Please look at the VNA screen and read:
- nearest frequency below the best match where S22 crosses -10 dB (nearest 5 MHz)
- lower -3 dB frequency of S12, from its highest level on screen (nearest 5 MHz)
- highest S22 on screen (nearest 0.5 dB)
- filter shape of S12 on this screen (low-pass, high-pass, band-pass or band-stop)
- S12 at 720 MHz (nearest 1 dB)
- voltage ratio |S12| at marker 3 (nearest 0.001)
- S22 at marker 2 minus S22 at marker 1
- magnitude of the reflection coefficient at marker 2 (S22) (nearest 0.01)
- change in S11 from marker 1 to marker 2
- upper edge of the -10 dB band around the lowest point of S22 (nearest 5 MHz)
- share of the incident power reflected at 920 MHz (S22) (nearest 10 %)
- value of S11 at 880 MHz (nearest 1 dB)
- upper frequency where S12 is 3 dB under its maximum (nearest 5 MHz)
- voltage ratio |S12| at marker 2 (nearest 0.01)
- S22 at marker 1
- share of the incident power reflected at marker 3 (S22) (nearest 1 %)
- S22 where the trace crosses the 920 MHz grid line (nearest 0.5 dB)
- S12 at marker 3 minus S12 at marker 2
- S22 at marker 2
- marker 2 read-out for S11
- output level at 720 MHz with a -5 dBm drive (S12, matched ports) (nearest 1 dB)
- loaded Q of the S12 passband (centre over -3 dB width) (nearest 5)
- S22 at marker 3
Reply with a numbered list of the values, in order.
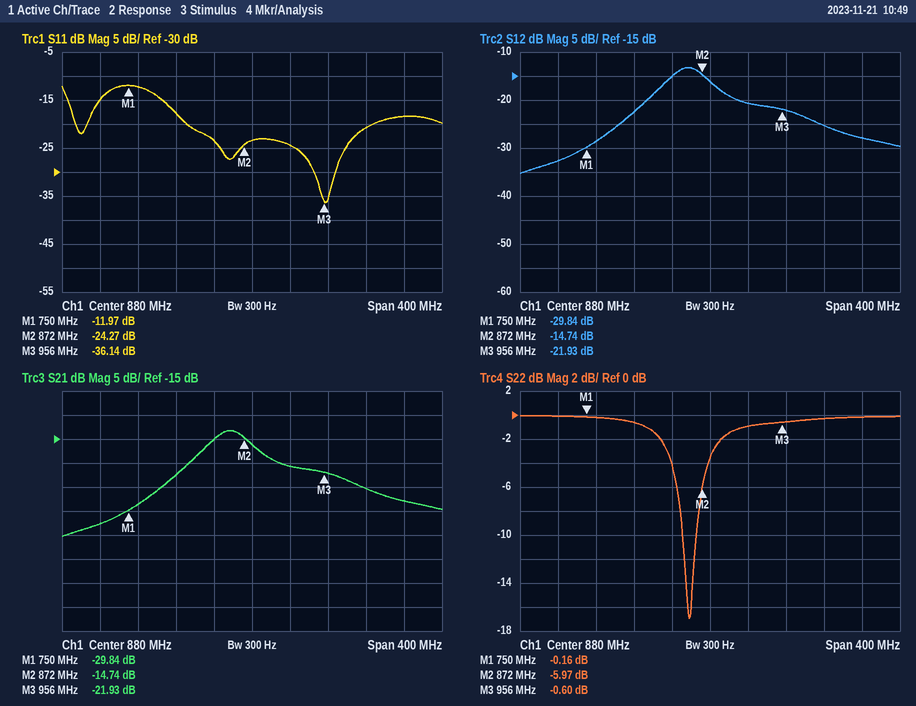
1. 850 MHz
2. 835 MHz
3. 0.0 dB
4. band-pass
5. -33 dB
6. 0.080
7. -5.81 dB
8. 0.50
9. -12.30 dB
10. 865 MHz
11. 80 %
12. -23 dB
13. 880 MHz
14. 0.18
15. -0.16 dB
16. 87 %
17. -1.0 dB
18. -7.19 dB
19. -5.97 dB
20. -24.27 dB
21. -38 dBm
22. 20
23. -0.60 dB
